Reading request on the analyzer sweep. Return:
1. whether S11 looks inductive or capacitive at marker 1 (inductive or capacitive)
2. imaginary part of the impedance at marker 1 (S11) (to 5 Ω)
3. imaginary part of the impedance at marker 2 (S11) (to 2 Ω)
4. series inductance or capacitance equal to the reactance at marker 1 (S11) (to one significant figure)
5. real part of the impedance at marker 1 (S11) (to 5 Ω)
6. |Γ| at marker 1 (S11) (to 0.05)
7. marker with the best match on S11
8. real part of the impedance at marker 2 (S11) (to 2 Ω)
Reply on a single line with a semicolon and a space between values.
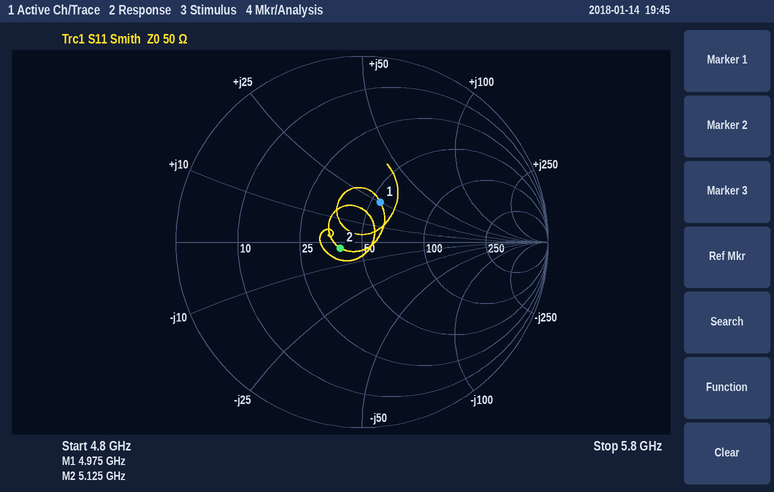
inductive; +25 Ω; -2 Ω; 800 pH; 55 Ω; 0.25; marker 2; 40 Ω
